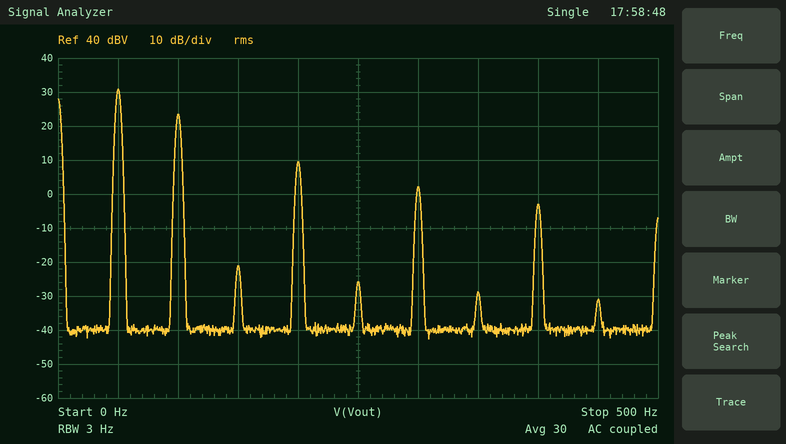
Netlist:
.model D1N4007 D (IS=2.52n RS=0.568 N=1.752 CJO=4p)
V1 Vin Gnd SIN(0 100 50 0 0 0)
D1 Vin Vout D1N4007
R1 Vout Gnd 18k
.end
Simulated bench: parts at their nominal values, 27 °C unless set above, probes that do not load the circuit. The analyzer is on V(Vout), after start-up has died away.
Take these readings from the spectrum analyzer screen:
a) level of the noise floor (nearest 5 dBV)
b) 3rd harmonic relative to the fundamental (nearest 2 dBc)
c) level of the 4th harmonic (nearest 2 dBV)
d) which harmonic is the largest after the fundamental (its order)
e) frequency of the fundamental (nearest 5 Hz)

-40 dBV
-52 dBc
10 dBV
2
50 Hz
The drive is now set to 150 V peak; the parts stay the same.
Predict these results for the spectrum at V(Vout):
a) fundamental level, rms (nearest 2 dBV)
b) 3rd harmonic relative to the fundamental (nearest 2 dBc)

34 dBV
-56 dBc
